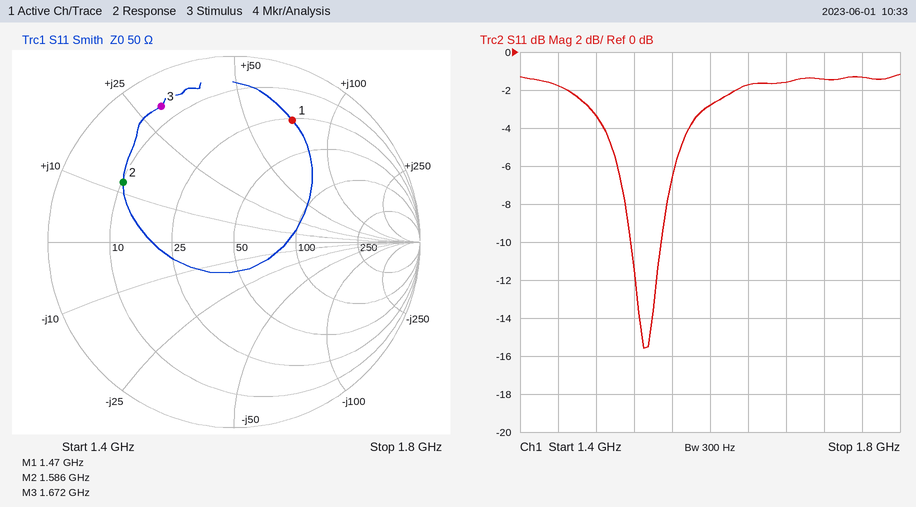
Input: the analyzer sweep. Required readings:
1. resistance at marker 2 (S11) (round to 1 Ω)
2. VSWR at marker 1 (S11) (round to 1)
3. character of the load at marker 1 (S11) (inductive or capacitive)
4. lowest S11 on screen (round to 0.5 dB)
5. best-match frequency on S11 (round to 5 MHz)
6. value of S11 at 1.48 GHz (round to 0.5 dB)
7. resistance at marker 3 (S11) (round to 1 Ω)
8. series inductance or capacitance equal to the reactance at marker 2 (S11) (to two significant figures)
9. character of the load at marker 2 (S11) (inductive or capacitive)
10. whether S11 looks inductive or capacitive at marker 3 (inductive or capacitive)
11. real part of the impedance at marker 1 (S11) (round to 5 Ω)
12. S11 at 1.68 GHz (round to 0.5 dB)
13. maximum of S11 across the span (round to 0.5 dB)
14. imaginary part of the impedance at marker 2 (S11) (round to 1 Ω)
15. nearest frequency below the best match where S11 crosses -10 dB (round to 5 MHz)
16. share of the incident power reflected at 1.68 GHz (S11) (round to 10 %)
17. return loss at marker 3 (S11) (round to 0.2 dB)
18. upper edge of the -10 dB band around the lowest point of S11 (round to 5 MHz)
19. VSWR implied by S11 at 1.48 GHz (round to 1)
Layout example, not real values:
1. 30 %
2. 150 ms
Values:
1. 10 Ω
2. 6
3. inductive
4. -15.5 dB
5. 1.530 GHz
6. -3.5 dB
7. 6 Ω
8. 1.2 nH
9. inductive
10. inductive
11. 25 Ω
12. -1.5 dB
13. -1.0 dB
14. +12 Ω
15. 1.515 GHz
16. 70 %
17. 1.6 dB
18. 1.550 GHz
19. 5
